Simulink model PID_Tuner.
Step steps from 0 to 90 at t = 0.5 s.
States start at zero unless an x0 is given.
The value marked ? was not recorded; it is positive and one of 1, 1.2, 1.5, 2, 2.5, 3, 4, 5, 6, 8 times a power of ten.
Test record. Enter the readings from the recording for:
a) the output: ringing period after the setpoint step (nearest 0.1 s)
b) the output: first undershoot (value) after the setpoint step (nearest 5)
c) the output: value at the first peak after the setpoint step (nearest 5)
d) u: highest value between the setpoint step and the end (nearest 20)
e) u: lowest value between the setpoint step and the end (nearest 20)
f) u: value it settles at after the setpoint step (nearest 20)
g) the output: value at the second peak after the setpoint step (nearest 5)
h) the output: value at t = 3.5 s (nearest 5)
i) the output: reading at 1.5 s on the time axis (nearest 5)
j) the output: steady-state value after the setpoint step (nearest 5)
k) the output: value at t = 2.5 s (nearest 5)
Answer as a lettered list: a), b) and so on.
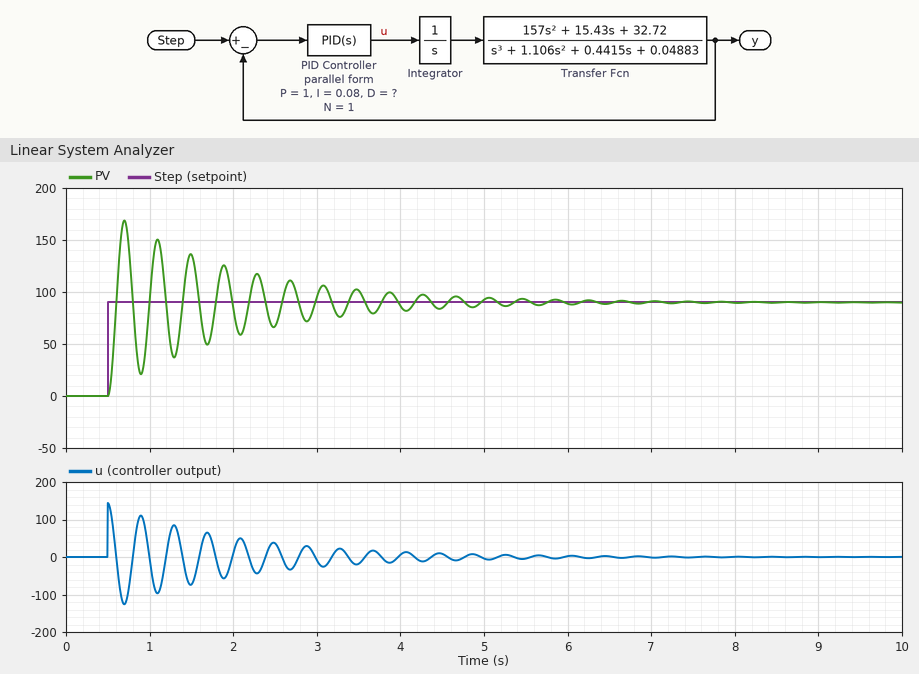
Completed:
a) 0.4 s
b) 20
c) 170
d) 140
e) -120
f) 0
g) 150
h) 100
i) 135
j) 90
k) 65
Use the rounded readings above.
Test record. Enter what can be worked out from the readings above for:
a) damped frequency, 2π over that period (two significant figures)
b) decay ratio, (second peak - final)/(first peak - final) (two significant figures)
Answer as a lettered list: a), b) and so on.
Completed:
a) 16 rad/s
b) 0.75
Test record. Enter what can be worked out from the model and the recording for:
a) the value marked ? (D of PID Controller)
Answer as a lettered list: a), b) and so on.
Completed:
a) 0.6
